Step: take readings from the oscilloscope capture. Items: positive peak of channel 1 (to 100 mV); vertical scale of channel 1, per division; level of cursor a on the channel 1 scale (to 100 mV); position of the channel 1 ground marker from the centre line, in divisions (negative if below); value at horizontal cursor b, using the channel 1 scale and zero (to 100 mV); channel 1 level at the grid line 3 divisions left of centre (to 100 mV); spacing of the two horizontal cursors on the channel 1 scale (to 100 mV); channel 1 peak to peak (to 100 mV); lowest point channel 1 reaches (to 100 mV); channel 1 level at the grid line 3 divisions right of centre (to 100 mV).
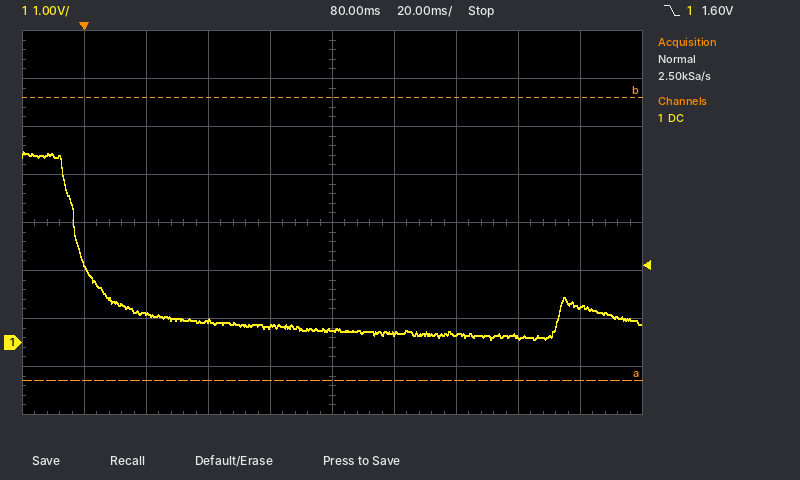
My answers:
4.0 V
1 V
-800 mV
-2.5 div
5.1 V
600 mV
5.9 V
3.9 V
100 mV
100 mV
